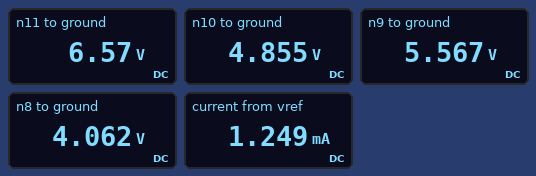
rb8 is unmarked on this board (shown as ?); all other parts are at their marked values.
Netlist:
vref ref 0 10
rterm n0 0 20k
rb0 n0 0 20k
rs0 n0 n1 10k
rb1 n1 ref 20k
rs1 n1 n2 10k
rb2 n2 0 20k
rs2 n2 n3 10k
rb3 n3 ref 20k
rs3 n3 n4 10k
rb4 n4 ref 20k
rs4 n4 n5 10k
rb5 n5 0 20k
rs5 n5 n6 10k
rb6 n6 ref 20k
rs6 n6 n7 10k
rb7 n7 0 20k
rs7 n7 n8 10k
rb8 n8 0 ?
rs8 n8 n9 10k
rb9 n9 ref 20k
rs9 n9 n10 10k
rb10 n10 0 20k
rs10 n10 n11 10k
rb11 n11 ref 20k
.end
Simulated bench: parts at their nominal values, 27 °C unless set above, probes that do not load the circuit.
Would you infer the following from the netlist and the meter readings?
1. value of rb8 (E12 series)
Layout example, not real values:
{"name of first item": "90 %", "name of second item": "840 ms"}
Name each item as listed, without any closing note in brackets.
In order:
{"value of rb8": "33 kΩ"}
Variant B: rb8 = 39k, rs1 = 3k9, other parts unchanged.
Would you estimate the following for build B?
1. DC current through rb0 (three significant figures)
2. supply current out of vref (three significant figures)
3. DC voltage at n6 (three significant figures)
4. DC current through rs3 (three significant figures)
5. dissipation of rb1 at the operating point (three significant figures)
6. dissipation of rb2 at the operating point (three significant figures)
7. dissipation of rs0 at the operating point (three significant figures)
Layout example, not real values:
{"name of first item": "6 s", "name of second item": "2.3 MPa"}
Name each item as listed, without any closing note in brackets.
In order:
{"DC current through rb0": "116 µA", "supply current out of vref": "1.24 mA", "DC voltage at n6": "5.45 V", "DC current through rs3": "7.67 µA", "dissipation of rb1 at the operating point": "1.44 mW", "dissipation of rb2 at the operating point": "1.01 mW", "dissipation of rs0 at the operating point": "538 µW"}
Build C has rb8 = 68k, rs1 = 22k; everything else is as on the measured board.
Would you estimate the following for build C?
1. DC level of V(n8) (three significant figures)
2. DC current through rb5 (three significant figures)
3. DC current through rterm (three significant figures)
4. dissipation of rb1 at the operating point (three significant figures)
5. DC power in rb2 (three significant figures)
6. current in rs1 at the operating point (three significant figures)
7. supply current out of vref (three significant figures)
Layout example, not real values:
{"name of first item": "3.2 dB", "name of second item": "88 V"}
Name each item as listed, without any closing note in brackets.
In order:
{"DC level of V(n8)": "4.62 V", "DC current through rb5": "240 µA", "DC current through rterm": "120 µA", "dissipation of rb1 at the operating point": "1.35 mW", "DC power in rb2": "945 µW", "current in rs1 at the operating point": "20.4 µA", "supply current out of vref": "1.22 mA"}
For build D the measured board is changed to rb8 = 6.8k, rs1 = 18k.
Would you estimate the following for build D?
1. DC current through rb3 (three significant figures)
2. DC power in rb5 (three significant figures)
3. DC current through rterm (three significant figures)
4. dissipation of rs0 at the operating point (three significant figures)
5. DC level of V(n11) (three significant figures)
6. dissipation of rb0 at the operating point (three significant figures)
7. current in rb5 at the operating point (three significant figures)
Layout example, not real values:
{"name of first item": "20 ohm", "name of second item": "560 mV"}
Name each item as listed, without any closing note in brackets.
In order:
{"DC current through rb3": "188 µA", "DC power in rb5": "1.01 mW", "DC current through rterm": "119 µA", "dissipation of rs0 at the operating point": "566 µW", "DC level of V(n11)": "6.21 V", "dissipation of rb0 at the operating point": "283 µW", "current in rb5 at the operating point": "224 µA"}
